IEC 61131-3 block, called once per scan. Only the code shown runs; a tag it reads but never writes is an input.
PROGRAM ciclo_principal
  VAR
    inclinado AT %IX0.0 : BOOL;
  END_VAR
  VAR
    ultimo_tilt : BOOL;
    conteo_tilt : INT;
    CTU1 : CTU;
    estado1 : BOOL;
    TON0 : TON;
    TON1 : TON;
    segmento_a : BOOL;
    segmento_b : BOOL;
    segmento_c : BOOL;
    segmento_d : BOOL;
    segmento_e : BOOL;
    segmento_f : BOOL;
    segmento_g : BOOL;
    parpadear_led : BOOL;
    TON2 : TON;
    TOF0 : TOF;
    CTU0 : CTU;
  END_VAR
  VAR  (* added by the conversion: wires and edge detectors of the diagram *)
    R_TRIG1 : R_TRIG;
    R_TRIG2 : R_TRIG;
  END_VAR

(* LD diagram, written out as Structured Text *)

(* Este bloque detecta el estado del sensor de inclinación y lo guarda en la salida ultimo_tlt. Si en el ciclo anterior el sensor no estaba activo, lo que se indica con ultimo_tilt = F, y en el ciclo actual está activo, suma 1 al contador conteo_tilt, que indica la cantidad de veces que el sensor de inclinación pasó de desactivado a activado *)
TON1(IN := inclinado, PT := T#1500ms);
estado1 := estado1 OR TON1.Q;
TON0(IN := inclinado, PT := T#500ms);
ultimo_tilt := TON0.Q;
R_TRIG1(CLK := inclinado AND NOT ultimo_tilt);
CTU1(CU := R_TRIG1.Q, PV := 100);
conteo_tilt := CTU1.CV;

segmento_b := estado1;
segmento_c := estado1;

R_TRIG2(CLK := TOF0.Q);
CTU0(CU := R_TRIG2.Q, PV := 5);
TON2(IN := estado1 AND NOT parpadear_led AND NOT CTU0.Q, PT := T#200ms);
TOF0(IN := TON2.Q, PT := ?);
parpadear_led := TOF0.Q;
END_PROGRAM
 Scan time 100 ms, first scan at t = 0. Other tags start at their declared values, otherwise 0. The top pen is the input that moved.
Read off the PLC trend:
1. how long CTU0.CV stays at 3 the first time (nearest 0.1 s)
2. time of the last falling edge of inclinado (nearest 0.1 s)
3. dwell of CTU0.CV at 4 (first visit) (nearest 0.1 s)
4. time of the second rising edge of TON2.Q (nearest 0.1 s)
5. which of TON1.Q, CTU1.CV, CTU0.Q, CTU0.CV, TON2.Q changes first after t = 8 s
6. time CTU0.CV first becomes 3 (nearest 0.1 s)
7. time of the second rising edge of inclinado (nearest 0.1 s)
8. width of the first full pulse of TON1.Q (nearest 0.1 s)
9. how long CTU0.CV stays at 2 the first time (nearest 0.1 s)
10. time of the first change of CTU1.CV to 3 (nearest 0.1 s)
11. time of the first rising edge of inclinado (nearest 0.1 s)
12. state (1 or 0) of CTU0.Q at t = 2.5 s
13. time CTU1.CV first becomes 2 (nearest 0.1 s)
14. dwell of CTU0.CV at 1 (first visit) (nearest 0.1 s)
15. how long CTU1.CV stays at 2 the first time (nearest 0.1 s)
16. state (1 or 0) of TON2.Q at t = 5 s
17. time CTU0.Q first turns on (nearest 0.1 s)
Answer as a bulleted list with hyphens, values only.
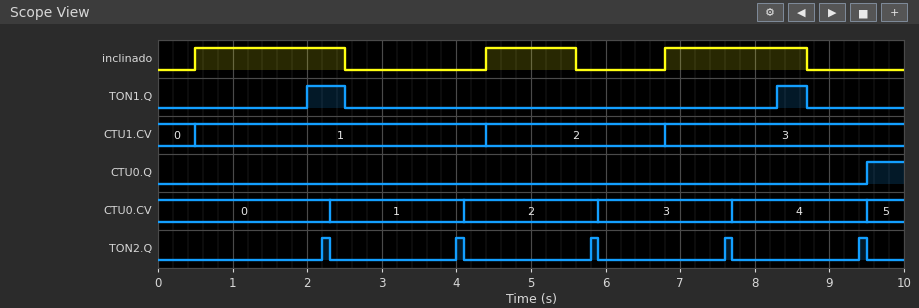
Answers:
- 1.8 s
- 8.7 s
- 1.8 s
- 4.0 s
- TON1.Q
- 5.9 s
- 4.4 s
- 0.5 s
- 1.8 s
- 6.8 s
- 0.5 s
- 0
- 4.4 s
- 1.8 s
- 2.4 s
- 0
- 9.5 s
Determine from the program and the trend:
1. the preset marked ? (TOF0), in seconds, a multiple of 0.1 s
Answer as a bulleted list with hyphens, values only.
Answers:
- 1.4 s
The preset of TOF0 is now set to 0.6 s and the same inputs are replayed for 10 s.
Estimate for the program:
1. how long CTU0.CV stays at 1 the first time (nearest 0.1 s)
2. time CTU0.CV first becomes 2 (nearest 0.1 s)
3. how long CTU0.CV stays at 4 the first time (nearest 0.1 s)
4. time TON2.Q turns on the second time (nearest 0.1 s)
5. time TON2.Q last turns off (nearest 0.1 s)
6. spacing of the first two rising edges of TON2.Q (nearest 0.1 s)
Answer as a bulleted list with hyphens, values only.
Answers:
- 1.0 s
- 3.3 s
- 1.0 s
- 3.2 s
- 6.3 s
- 1.0 s
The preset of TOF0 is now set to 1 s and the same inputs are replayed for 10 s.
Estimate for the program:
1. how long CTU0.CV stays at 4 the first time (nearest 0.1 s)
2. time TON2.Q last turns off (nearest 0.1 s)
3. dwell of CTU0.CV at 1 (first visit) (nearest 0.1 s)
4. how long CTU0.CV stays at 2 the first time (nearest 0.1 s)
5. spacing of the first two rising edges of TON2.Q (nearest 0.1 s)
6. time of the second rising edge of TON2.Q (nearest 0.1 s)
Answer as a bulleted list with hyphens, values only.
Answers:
- 1.4 s
- 7.9 s
- 1.4 s
- 1.4 s
- 1.4 s
- 3.6 s
